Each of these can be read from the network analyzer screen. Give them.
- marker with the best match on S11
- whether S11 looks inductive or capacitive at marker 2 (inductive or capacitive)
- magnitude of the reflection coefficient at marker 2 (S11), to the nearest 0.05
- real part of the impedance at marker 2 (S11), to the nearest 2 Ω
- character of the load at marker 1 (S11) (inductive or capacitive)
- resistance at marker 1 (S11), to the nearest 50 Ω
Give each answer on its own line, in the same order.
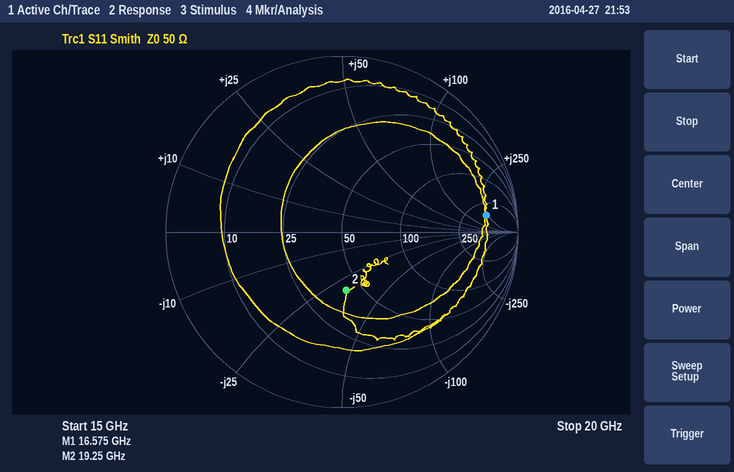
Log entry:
marker 2
capacitive
0.35
42 Ω
inductive
400 Ω
